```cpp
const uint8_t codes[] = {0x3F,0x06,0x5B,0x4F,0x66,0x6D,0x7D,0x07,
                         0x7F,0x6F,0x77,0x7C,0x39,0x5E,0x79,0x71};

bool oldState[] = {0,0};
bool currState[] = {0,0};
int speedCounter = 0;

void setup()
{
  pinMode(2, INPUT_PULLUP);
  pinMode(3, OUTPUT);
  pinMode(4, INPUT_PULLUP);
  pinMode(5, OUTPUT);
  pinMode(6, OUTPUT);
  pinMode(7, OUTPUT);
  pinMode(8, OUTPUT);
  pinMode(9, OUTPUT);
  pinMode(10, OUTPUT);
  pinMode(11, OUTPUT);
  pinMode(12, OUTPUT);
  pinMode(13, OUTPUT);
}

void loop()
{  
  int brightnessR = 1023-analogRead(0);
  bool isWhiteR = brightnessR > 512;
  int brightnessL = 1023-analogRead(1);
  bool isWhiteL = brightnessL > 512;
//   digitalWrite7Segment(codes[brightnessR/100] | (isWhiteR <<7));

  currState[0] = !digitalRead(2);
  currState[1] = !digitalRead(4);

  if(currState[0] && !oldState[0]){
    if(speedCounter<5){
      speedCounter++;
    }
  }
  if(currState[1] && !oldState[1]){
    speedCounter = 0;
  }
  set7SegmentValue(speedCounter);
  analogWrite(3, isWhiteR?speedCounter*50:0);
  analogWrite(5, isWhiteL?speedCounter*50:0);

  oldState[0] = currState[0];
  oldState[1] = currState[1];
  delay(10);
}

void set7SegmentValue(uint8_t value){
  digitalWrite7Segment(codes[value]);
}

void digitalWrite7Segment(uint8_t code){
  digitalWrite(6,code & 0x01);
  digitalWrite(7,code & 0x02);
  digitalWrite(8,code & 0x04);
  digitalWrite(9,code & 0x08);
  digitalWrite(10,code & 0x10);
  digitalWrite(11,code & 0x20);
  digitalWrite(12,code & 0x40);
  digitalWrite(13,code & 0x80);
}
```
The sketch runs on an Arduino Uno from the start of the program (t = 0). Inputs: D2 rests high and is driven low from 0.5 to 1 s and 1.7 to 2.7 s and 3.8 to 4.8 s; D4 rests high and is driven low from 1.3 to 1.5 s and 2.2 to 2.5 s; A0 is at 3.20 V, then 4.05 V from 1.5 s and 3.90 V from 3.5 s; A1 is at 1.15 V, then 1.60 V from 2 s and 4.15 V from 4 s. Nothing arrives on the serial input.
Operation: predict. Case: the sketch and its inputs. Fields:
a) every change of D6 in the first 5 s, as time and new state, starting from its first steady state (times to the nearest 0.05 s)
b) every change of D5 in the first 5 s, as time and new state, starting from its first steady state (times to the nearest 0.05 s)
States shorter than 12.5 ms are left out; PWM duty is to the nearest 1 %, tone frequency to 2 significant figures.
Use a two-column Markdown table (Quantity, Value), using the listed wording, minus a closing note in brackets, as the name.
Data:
| Quantity | Value |
|---|---|
| every change of D6 in the first 5 s, as time and new state, starting from its first steady state | 0 s high; 0.5 s low; 1.3 s high; 1.7 s low; 2.2 s high; 3.8 s low |
| every change of D5 in the first 5 s, as time and new state, starting from its first steady state | 0 s low; 0.5 s PWM 20 %; 1.3 s low; 1.7 s PWM 20 %; 2.2 s low; 3.8 s PWM 20 %; 4 s low |
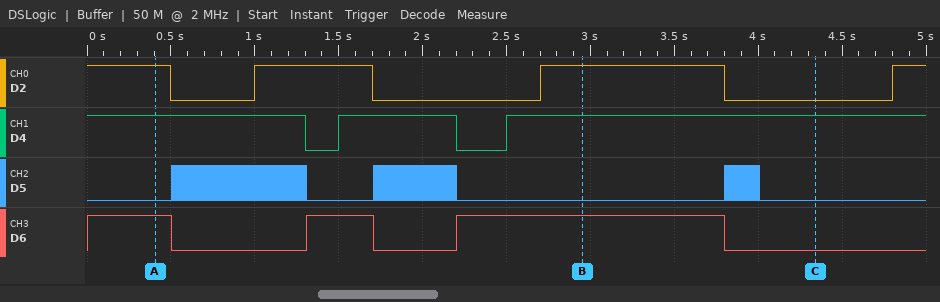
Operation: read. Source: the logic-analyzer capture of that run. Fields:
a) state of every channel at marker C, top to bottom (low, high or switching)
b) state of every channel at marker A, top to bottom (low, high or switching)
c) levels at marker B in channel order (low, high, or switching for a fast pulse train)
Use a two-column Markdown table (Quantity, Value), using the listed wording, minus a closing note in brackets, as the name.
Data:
| Quantity | Value |
|---|---|
| state of every channel at marker C, top to bottom | D2 low, D4 high, D5 low, D6 low |
| state of every channel at marker A, top to bottom | D2 high, D4 high, D5 low, D6 high |
| levels at marker B in channel order | D2 high, D4 high, D5 low, D6 high |
